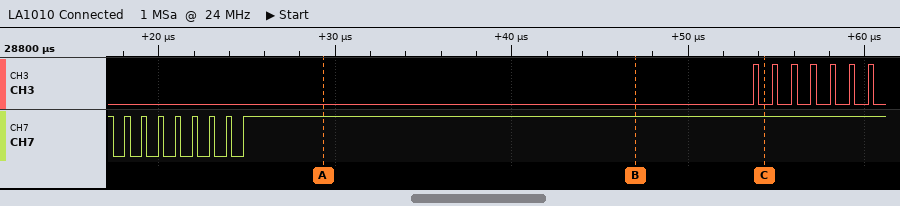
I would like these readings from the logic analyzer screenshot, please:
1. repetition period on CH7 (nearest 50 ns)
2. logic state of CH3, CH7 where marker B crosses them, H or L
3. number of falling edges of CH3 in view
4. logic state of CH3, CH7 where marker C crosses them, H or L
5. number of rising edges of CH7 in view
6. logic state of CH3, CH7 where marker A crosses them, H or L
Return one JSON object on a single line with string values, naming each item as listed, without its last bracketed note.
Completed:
{"repetition period on CH7": "950 ns", "logic state of CH3, CH7 where marker B crosses them, H or L": "CH3=L, CH7=H", "number of falling edges of CH3 in view": "7", "logic state of CH3, CH7 where marker C crosses them, H or L": "CH3=L, CH7=H", "number of rising edges of CH7 in view": "8", "logic state of CH3, CH7 where marker A crosses them, H or L": "CH3=L, CH7=H"}
